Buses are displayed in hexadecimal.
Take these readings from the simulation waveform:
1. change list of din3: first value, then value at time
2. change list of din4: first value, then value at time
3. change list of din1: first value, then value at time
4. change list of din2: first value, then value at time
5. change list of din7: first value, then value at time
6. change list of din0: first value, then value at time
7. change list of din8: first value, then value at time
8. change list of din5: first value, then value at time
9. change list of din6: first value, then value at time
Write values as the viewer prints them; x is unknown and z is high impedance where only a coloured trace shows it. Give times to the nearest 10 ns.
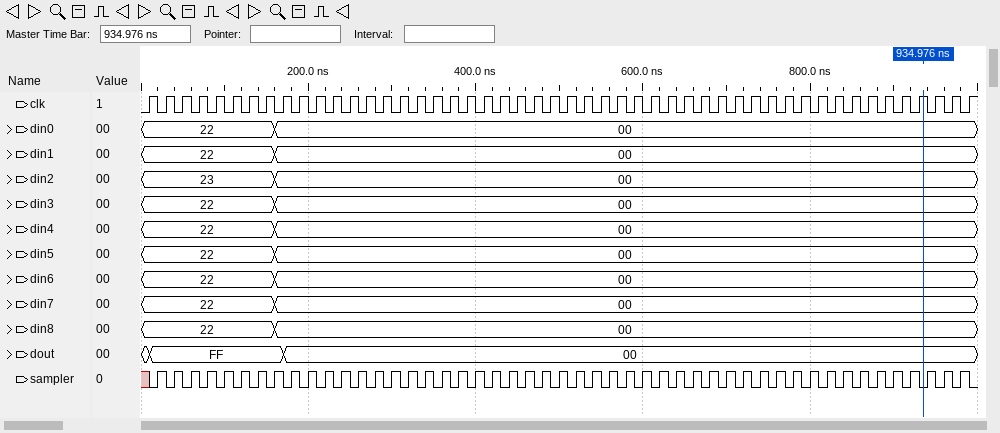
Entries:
22, 00 at 160 ns
22, 00 at 160 ns
22, 00 at 160 ns
23, 00 at 160 ns
22, 00 at 160 ns
22, 00 at 160 ns
22, 00 at 160 ns
22, 00 at 160 ns
22, 00 at 160 ns
